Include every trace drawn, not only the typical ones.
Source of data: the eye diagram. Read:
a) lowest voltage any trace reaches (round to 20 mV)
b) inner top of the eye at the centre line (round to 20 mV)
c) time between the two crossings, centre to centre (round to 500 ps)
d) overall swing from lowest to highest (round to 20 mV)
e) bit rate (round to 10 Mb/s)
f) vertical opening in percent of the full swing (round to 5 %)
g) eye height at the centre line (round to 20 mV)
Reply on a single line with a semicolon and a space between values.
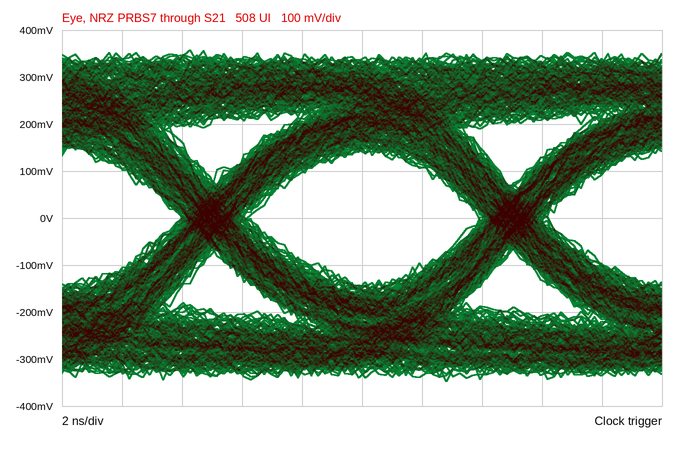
-340 mV; 140 mV; 10.0 ns; 700 mV; 100 Mb/s; 40 %; 280 mV
